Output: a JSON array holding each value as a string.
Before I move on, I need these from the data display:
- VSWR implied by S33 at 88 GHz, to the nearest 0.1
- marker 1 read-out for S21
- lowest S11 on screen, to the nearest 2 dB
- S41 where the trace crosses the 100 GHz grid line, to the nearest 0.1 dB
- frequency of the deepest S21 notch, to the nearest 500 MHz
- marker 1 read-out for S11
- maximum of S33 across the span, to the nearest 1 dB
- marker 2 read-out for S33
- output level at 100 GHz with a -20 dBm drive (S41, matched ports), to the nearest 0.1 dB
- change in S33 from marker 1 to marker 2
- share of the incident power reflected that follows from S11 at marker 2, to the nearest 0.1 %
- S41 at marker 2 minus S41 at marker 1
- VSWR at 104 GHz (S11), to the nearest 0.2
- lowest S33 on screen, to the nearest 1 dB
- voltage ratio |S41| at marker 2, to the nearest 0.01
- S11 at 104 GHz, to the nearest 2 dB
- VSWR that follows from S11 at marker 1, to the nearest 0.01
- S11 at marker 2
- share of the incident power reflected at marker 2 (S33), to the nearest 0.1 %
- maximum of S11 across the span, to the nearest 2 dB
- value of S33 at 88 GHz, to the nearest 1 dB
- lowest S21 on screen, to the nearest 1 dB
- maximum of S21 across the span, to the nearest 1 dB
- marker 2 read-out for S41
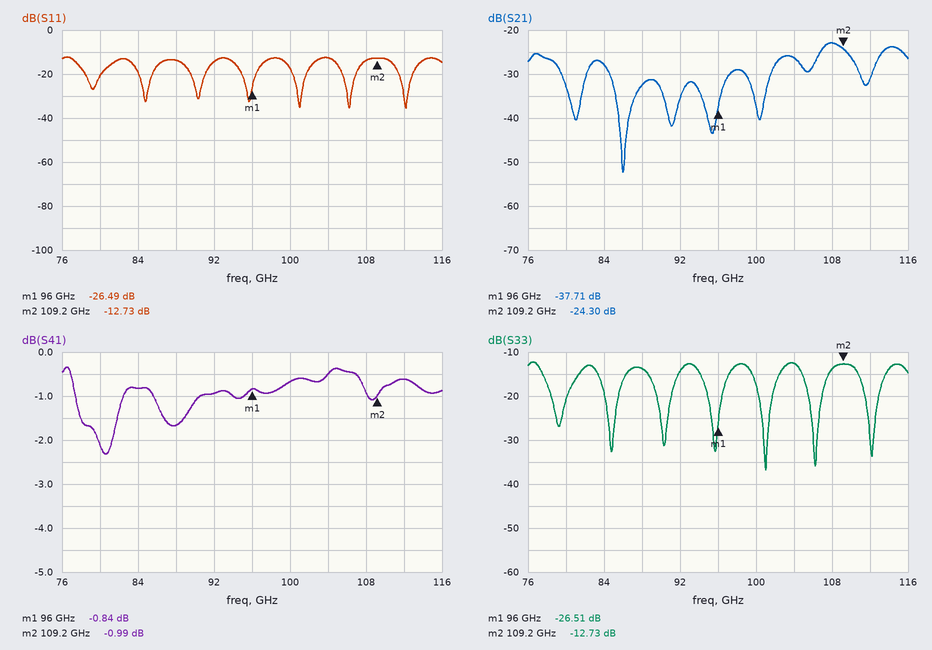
["1.5", "-37.71 dB", "-36 dB", "-0.7 dB", "86.0 GHz", "-26.49 dB", "-12 dB", "-12.73 dB", "-20.7 dBm", "13.78 dB", "5.3 %", "-0.15 dB", "1.6", "-37 dB", "0.89", "-12 dB", "1.10", "-12.73 dB", "5.3 %", "-12 dB", "-14 dB", "-52 dB", "-23 dB", "-0.99 dB"]
